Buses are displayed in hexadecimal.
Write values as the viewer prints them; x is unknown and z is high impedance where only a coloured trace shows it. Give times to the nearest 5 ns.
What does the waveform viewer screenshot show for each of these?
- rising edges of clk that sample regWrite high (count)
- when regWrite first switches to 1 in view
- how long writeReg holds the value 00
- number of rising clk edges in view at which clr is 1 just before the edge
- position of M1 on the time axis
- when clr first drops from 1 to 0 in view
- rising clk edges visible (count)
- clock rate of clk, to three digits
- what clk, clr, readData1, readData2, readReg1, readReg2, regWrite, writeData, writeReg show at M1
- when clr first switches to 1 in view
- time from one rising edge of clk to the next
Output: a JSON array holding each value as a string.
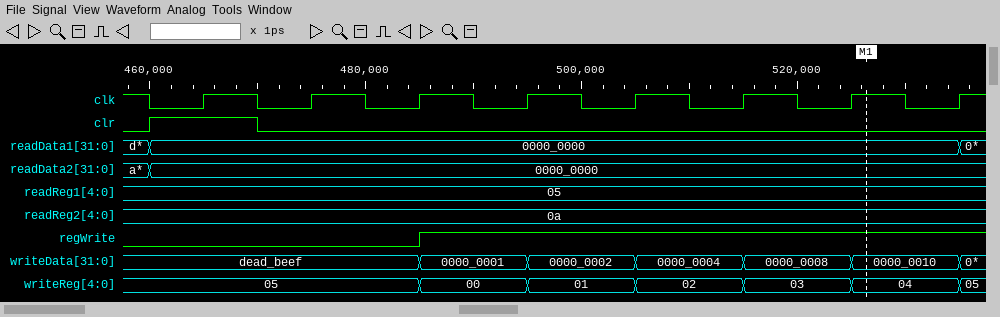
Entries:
["5", "485 ns", "10 ns", "1", "525 ns", "470 ns", "8", "100 MHz", "clk=1, clr=0, readData1=0000_0000, readData2=0000_0000, readReg1=05, readReg2=0a, regWrite=1, writeData=0000_0010, writeReg=04", "460 ns", "10 ns"]
